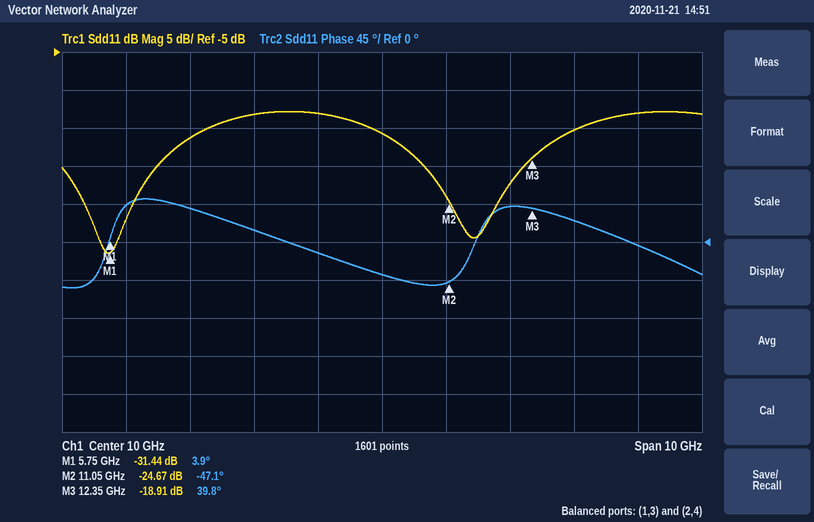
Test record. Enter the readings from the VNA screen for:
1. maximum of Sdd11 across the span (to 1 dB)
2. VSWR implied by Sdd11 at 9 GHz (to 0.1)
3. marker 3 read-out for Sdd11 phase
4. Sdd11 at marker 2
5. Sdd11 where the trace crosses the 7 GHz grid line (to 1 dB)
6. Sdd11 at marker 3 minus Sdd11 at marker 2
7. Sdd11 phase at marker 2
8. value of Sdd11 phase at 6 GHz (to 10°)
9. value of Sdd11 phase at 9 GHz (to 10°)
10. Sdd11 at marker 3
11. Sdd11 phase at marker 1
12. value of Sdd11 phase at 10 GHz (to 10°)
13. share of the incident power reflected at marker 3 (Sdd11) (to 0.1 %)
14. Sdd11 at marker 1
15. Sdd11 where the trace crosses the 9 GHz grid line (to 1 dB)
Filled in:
-13 dB
1.6
39.8°
-24.67 dB
-16 dB
5.76 dB
-47.1°
40°
-10°
-18.91 dB
3.9°
-40°
1.3 %
-31.44 dB
-13 dB
